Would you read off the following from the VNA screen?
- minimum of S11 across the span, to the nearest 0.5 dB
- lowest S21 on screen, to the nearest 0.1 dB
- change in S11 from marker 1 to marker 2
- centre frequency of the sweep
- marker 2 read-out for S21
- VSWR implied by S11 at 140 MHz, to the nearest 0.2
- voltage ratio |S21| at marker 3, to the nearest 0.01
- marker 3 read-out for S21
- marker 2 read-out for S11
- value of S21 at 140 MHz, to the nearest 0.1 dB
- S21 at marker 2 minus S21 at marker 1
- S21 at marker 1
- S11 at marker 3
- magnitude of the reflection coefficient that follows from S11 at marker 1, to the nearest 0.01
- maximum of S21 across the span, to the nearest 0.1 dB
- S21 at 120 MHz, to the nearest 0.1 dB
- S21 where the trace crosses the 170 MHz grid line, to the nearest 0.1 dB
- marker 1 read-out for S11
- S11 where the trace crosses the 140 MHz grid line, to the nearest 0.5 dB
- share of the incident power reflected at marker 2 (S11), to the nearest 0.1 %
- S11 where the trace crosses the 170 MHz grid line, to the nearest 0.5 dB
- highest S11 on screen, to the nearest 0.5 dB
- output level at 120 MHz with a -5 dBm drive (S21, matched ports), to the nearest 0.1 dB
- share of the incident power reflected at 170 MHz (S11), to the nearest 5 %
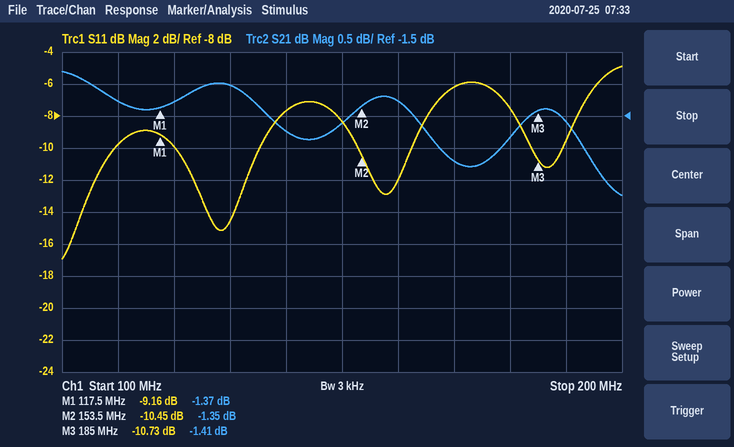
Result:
-17.0 dB
-2.7 dB
-1.29 dB
150 MHz
-1.35 dB
2.4
0.85
-1.41 dB
-10.45 dB
-1.7 dB
0.02 dB
-1.37 dB
-10.73 dB
0.35
-0.8 dB
-1.3 dB
-2.2 dB
-9.16 dB
-7.5 dB
9.0 %
-6.0 dB
-5.0 dB
-6.3 dBm
25 %
